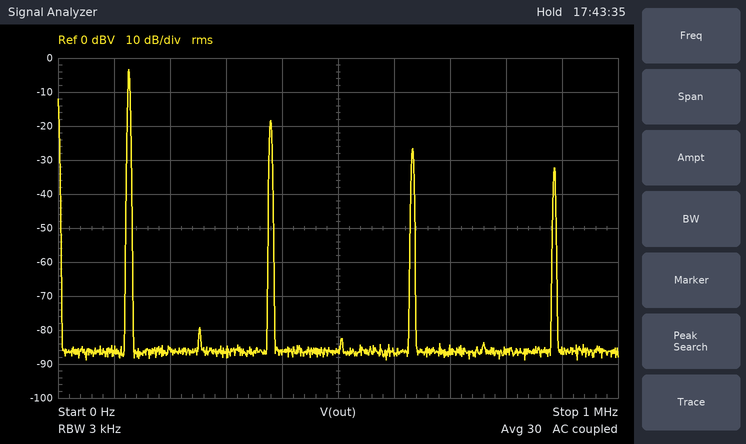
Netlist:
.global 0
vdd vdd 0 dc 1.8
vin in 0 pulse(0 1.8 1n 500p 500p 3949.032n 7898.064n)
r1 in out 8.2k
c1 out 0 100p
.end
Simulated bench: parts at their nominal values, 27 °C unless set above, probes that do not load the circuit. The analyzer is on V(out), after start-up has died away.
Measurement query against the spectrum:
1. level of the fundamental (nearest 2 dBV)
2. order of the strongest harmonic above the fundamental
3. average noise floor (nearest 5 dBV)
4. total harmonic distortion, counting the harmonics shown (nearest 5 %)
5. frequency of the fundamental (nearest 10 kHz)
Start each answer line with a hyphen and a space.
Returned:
- -4 dBV
- 3
- -85 dBV
- 20 %
- 130 kHz
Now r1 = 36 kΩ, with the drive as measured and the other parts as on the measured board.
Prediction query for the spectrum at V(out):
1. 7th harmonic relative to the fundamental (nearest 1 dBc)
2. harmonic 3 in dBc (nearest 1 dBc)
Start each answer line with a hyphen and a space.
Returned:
- -33 dBc
- -19 dBc
